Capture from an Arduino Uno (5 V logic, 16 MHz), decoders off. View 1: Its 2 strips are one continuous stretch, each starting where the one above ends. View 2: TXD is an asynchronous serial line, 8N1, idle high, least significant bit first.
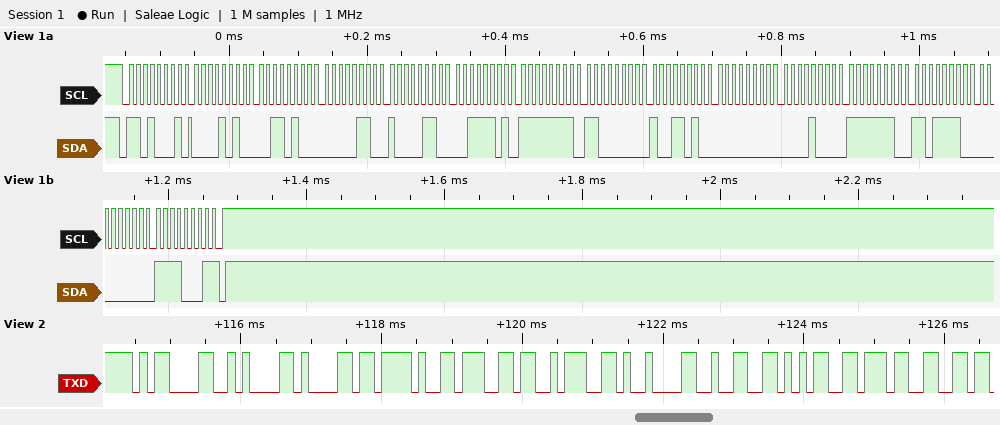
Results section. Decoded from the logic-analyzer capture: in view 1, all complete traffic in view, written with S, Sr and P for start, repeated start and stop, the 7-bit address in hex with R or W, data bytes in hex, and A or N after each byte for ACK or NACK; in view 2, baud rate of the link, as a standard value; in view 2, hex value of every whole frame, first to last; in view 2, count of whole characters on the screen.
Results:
S 68R A 0A A 34 A 06 A 86 A 3D A FF A C0 A 9A A 00 A 08 A FE A DE A 00 A F1 N P
9600 baud
0D 0A 61 2F 67 3A 09 32 35 37
10
